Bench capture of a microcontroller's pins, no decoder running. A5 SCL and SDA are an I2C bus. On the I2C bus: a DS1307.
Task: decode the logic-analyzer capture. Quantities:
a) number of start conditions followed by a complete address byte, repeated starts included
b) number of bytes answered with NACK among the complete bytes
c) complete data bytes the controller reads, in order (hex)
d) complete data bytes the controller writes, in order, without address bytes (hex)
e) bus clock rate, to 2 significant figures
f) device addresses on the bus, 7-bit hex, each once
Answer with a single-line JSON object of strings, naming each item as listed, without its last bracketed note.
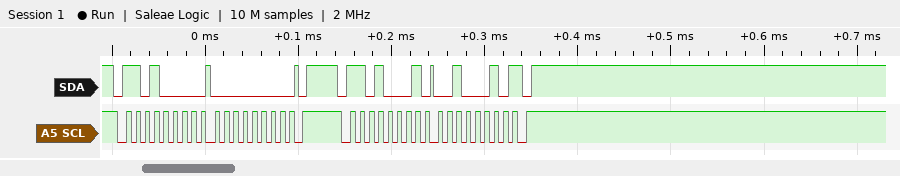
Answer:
{"number of start conditions followed by a complete address byte, repeated starts included": "2", "number of bytes answered with NACK among the complete bytes": "1", "complete data bytes the controller reads, in order": "22", "complete data bytes the controller writes, in order, without address bytes": "00", "bus clock rate, to 2 significant figures": "100 kHz", "device addresses on the bus, 7-bit hex, each once": "0x68"}
